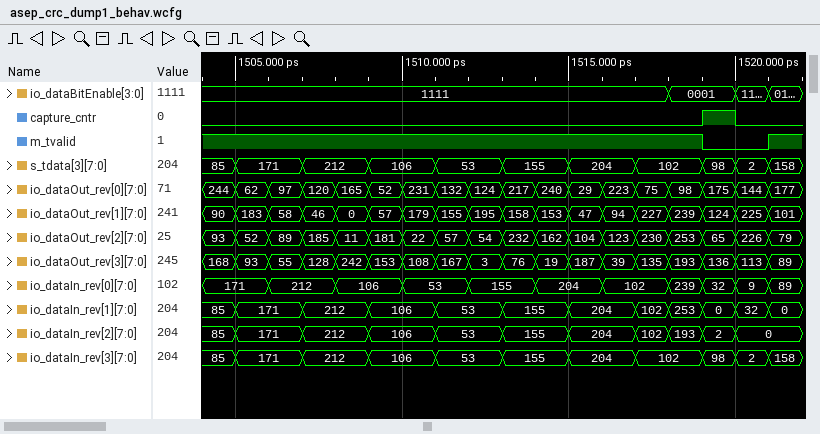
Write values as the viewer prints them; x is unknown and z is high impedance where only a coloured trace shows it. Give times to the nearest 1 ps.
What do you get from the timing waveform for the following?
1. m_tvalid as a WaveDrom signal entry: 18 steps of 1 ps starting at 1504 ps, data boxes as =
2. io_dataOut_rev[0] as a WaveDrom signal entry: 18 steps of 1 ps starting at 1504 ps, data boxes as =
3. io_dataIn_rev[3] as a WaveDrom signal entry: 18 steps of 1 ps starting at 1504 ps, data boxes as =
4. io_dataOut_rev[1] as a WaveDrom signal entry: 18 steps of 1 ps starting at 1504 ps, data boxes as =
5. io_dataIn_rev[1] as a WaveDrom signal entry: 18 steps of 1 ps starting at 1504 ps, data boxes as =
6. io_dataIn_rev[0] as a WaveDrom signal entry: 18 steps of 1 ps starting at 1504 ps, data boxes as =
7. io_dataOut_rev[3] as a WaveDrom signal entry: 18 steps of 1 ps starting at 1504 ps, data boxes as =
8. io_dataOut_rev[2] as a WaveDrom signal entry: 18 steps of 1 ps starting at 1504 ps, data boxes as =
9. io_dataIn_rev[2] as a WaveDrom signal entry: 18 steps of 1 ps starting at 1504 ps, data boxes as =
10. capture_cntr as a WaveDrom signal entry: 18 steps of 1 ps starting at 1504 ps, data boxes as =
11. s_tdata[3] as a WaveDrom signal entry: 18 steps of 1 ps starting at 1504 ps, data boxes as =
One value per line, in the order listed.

{name: 'm_tvalid', wave: '1..............0.1'}
{name: 'io_dataOut_rev[0]', wave: '==================', data: '244 62 97 120 165 52 231 132 124 217 240 29 223 75 98 175 144 177'}
{name: 'io_dataIn_rev[3]', wave: '==.=.=.=.=.=.=.===', data: '85 171 212 106 53 155 204 102 98 2 158'}
{name: 'io_dataOut_rev[1]', wave: '==================', data: '90 183 58 46 0 57 179 155 195 158 153 47 94 227 239 124 225 101'}
{name: 'io_dataIn_rev[1]', wave: '==.=.=.=.=.=.=====', data: '85 171 212 106 53 155 204 102 253 0 32 0'}
{name: 'io_dataIn_rev[0]', wave: '=.=.=.=.=.=.=.====', data: '171 212 106 53 155 204 102 239 32 9 89'}
{name: 'io_dataOut_rev[3]', wave: '==================', data: '168 93 55 128 242 153 108 167 3 76 19 187 39 135 193 136 113 89'}
{name: 'io_dataOut_rev[2]', wave: '==================', data: '93 52 89 185 11 181 22 57 54 232 162 104 123 230 253 65 226 79'}
{name: 'io_dataIn_rev[2]', wave: '==.=.=.=.=.=.====.', data: '85 171 212 106 53 155 204 102 193 2 0'}
{name: 'capture_cntr', wave: '0..............10.'}
{name: 's_tdata[3]', wave: '==.=.=.=.=.=.=.===', data: '85 171 212 106 53 155 204 102 98 2 158'}
